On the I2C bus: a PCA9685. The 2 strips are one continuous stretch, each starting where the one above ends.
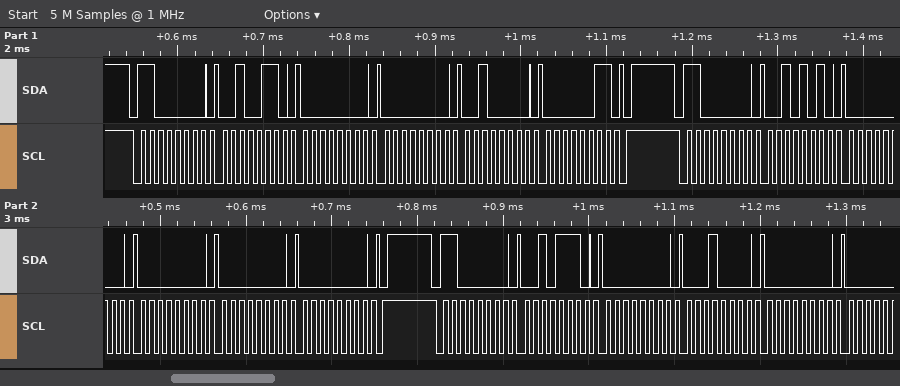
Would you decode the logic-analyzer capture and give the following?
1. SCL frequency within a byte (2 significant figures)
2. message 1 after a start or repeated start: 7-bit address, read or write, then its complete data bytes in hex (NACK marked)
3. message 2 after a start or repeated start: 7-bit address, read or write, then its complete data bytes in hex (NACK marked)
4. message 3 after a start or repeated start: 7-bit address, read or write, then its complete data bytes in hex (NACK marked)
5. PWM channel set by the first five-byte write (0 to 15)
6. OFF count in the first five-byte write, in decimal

100 kHz
0x60 write: 26 00 00 20 03
0x60 write: 2A 00 00 00 00
0x60 write: 2E 00 10 00
8
800
